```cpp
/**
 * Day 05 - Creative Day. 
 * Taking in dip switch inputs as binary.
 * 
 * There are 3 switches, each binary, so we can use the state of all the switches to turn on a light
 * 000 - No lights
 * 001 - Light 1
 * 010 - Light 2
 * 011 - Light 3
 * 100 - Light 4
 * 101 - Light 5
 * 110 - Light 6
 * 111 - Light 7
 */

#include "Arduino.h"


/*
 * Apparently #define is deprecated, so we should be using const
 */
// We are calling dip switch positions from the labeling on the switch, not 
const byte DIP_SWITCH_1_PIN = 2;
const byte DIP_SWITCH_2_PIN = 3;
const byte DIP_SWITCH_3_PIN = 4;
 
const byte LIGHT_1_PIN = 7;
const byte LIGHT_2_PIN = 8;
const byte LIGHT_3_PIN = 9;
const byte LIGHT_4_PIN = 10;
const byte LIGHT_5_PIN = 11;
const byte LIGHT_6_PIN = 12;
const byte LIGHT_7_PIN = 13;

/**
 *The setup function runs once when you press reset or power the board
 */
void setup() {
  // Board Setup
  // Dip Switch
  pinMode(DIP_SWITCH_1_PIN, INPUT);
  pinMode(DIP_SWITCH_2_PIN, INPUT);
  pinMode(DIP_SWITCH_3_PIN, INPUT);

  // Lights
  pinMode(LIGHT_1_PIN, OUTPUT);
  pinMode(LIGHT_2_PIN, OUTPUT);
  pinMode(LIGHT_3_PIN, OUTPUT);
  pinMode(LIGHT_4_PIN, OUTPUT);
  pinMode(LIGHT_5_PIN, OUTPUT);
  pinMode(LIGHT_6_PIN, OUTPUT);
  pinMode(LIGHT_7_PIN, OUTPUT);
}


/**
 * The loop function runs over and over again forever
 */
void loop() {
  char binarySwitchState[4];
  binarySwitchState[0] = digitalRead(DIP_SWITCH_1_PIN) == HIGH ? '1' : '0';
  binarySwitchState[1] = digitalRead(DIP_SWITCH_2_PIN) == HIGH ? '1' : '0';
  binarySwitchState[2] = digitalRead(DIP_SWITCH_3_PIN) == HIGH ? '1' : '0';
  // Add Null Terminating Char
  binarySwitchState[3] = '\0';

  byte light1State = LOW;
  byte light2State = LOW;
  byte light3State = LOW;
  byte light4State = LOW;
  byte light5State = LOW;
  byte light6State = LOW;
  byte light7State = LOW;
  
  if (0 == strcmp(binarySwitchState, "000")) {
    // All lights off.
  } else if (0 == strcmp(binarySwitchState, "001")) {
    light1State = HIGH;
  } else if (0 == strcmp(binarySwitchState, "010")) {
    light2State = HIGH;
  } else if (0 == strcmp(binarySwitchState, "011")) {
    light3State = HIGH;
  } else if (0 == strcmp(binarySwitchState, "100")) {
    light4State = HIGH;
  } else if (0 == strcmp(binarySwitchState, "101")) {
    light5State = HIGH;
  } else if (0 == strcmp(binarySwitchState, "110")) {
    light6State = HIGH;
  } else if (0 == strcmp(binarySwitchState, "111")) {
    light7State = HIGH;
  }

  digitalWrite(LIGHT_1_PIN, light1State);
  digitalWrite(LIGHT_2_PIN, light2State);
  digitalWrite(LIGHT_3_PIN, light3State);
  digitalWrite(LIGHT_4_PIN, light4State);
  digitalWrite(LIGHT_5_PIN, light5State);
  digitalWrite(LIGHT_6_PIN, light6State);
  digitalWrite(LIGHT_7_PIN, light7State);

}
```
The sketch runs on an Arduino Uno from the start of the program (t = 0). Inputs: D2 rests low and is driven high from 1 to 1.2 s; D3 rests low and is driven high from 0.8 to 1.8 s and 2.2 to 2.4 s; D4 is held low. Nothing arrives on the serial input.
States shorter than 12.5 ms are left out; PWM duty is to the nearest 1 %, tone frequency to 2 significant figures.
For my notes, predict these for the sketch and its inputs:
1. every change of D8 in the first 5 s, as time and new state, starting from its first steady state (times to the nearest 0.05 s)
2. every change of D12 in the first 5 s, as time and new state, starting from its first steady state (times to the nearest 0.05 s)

0 s low; 0.8 s high; 1 s low; 1.2 s high; 1.8 s low; 2.2 s high; 2.4 s low
0 s low; 1 s high; 1.2 s low
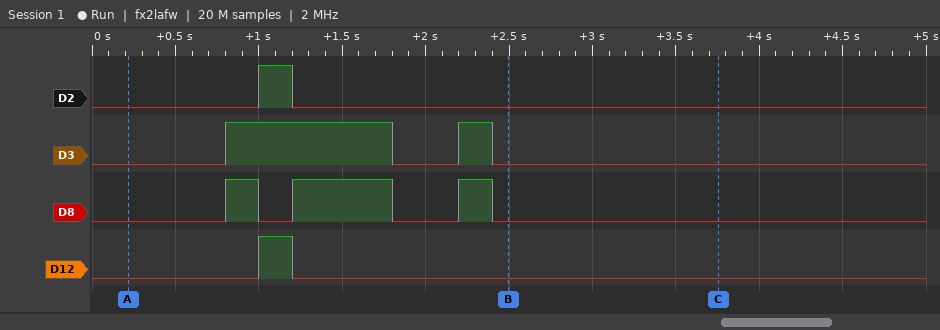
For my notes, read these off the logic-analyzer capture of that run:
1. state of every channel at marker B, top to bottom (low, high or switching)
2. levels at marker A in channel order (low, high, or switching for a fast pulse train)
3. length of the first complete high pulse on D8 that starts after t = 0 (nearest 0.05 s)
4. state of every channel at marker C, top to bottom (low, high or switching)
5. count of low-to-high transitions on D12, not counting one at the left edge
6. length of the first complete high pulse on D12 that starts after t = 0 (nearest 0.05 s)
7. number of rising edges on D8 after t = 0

D2 low, D3 low, D8 low, D12 low
D2 low, D3 low, D8 low, D12 low
0.20 s
D2 low, D3 low, D8 low, D12 low
1
0.20 s
3
